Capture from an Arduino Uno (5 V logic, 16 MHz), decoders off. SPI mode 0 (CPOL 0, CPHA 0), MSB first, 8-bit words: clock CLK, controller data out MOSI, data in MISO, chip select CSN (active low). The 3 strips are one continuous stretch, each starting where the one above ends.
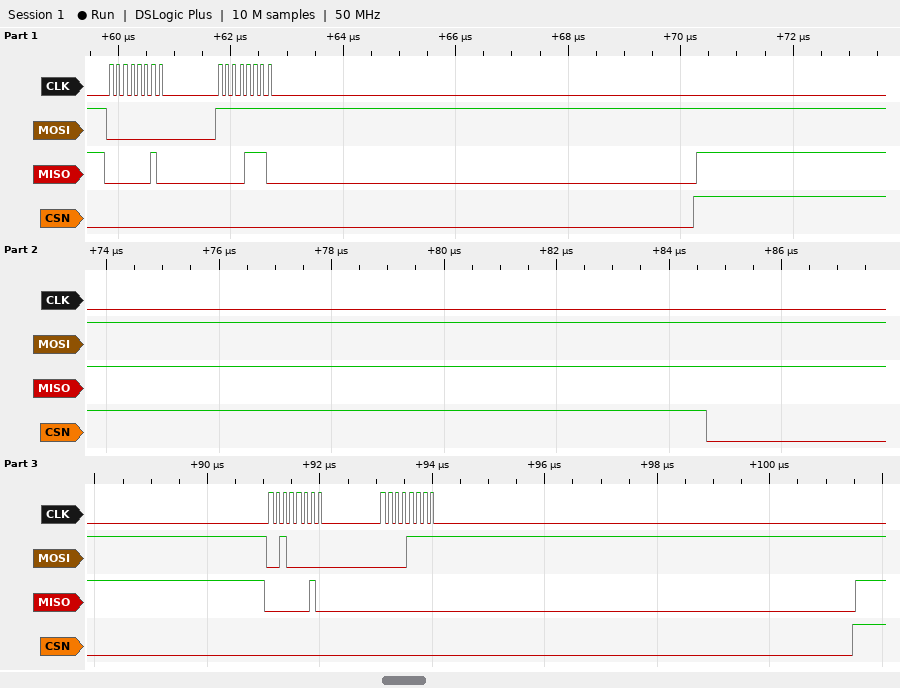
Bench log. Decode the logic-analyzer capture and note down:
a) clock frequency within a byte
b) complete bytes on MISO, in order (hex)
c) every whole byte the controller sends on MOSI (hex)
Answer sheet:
8 MHz
02 0E 02 00
00 FF 20 0F
